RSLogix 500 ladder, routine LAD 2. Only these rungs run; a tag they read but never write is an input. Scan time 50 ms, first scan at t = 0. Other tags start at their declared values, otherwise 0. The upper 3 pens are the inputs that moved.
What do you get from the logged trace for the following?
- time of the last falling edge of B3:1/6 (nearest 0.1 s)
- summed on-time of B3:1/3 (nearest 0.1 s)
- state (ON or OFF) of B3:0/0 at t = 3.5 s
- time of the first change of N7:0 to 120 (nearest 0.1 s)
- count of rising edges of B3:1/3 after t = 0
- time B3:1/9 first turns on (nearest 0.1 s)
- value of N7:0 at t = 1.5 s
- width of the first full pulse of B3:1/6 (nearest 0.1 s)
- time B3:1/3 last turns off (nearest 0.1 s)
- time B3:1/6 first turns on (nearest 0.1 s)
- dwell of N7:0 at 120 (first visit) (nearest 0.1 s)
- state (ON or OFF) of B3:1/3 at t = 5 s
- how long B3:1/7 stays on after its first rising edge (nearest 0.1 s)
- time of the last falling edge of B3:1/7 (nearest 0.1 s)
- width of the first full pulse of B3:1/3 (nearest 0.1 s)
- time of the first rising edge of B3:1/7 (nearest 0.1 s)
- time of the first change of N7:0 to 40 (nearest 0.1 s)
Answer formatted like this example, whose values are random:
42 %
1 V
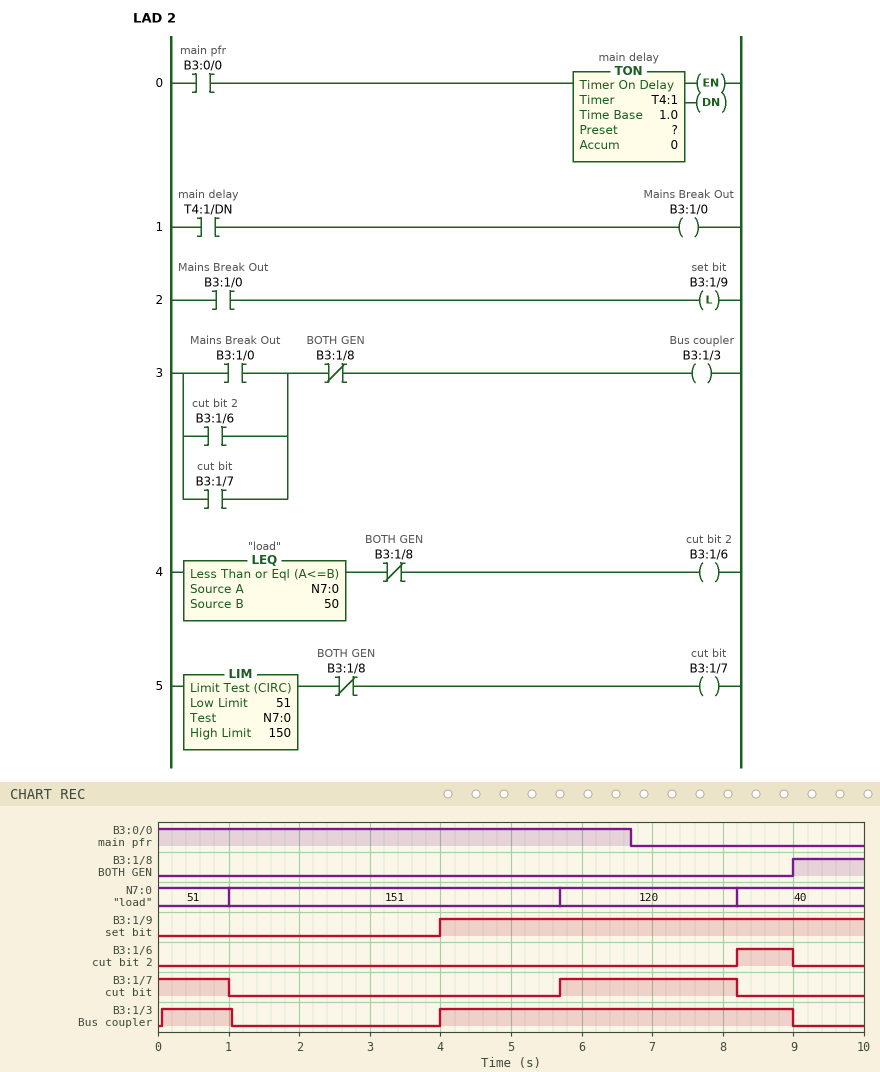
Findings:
9.0 s
6.0 s
ON
5.7 s
2
4.0 s
151
0.8 s
9.0 s
8.2 s
2.5 s
ON
2.5 s
8.2 s
1.0 s
5.7 s
8.2 s
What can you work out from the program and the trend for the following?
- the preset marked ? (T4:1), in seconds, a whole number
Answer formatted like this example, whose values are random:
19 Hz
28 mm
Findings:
4 s
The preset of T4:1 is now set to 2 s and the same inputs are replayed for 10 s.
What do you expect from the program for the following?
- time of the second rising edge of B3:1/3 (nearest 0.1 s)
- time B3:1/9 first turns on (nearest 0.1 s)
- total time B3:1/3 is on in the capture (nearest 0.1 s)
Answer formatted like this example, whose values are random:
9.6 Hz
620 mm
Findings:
2.0 s
2.0 s
8.0 s
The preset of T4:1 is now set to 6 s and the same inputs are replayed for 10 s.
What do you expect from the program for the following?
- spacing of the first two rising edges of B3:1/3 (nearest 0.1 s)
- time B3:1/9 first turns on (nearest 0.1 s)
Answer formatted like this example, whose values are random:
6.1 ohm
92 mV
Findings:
5.7 s
6.0 s
